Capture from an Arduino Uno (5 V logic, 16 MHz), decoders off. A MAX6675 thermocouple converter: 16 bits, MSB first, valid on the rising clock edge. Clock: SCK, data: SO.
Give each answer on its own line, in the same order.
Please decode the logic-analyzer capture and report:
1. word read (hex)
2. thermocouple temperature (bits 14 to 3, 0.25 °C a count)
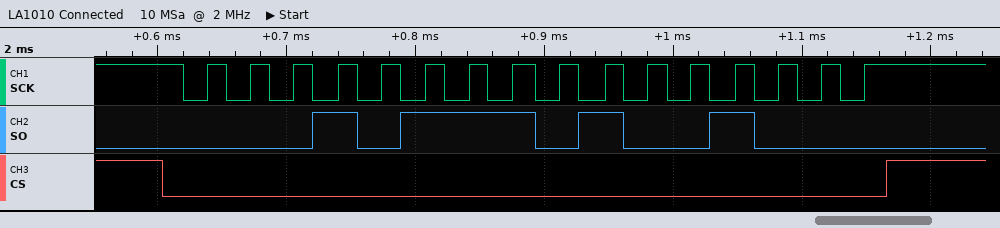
0x1748
186.25 °C
